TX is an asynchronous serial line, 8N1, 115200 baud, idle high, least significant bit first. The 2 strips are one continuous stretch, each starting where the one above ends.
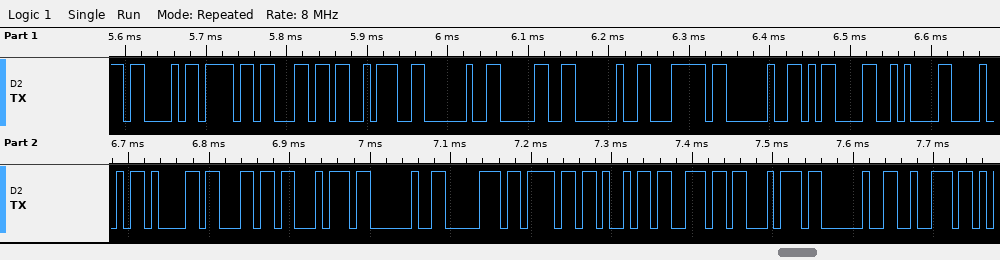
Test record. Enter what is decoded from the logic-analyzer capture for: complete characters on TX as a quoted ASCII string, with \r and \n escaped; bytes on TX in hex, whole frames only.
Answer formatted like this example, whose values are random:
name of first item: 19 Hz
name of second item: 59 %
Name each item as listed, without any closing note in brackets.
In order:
complete characters on TX as a quoted ASCII string, with \r and \n escaped: "Col: 0 | \r\nHalt point r"
bytes on TX in hex, whole frames only: 43 6F 6C 3A 20 30 20 7C 20 0D 0A 48 61 6C 74 20 70 6F 69 6E 74 20 72
